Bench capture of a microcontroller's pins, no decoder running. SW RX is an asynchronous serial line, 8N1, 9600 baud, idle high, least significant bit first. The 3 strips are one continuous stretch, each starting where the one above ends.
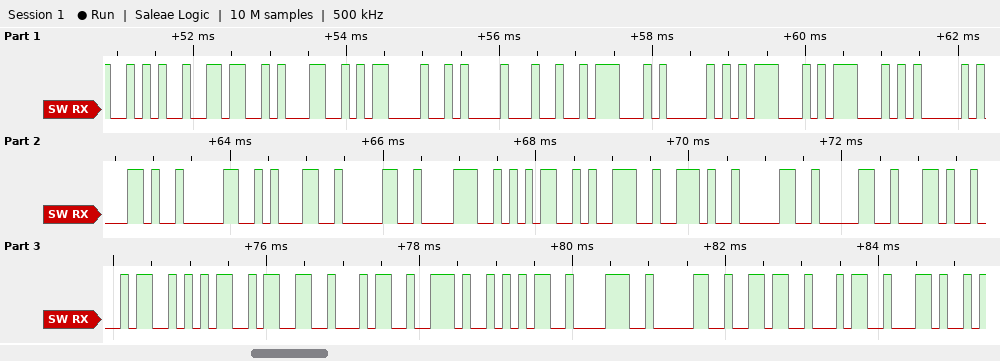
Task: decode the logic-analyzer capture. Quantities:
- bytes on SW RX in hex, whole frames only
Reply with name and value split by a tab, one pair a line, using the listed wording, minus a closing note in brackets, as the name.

bytes on SW RX in hex, whole frames only	0x2A 0x36 0x31 0x0D 0x0A 0x24 0x47 0x50 0x47 0x47 0x41 0x2C 0x30 0x31 0x30 0x38 0x35 0x39 0x2E 0x30 0x30 0x2C 0x34 0x35 0x33 0x34 0x2E 0x35 0x38 0x30 0x36 0x34 0x2C
